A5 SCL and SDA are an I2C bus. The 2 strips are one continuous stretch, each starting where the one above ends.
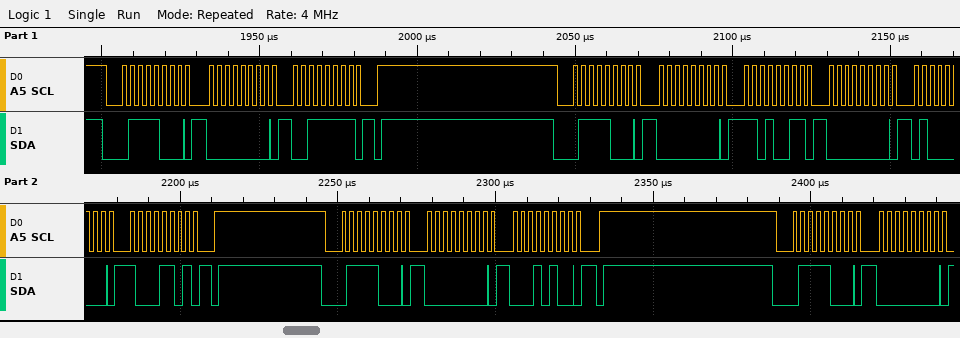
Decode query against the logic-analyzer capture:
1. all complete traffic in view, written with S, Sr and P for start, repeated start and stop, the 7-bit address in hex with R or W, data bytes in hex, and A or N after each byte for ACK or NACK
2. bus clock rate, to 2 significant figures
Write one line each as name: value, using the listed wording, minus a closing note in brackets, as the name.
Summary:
all complete traffic in view, written with S, Sr and P for start, repeated start and stop, the 7-bit address in hex with R or W, data bytes in hex, and A or N after each byte for ACK or NACK: S 3CW A 00 A 3F A P S 3CW A 00 A D3 A 00 A 40 A 8D A P S 3CW A 00 A 14 A P S 3CW A 00 A
bus clock rate, to 2 significant figures: 400 kHz
